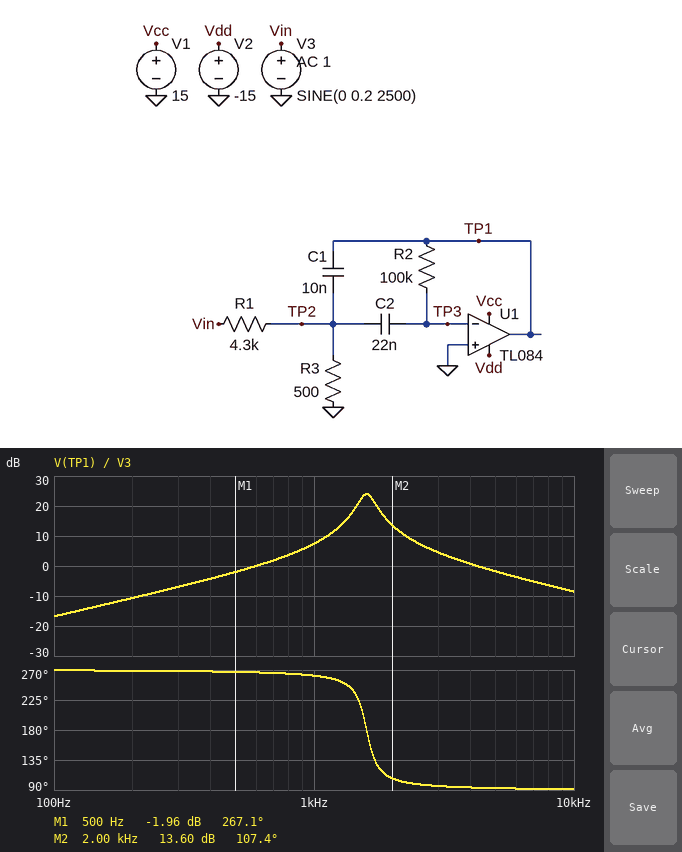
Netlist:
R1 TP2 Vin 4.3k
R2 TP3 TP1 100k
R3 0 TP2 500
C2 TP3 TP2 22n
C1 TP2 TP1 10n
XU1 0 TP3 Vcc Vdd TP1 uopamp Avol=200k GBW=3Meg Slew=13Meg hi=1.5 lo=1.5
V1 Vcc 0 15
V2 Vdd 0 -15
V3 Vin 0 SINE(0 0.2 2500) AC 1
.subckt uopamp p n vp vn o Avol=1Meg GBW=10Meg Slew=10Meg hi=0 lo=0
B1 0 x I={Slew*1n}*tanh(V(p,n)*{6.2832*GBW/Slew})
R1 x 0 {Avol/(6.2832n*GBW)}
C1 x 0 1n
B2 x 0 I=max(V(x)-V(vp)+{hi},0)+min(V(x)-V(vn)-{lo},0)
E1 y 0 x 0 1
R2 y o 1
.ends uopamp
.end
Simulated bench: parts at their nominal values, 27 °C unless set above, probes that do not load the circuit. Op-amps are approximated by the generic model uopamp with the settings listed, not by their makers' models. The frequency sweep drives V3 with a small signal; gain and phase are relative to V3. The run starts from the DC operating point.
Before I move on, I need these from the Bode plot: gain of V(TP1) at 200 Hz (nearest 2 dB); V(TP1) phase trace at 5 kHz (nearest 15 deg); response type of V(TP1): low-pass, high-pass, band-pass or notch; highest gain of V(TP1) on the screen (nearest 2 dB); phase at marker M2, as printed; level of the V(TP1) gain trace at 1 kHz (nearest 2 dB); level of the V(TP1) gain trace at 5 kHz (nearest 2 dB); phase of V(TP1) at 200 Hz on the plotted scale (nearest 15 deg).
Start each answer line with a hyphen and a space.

- -10 dB
- 90 deg
- band-pass
- 24 dB
- 107.4 deg
- 8 dB
- -2 dB
- 270 deg
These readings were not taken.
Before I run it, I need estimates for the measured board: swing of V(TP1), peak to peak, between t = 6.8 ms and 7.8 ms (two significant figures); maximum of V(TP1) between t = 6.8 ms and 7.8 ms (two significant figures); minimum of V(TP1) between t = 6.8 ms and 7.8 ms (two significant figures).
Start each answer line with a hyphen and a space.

- 980 mV
- 490 mV
- -490 mV
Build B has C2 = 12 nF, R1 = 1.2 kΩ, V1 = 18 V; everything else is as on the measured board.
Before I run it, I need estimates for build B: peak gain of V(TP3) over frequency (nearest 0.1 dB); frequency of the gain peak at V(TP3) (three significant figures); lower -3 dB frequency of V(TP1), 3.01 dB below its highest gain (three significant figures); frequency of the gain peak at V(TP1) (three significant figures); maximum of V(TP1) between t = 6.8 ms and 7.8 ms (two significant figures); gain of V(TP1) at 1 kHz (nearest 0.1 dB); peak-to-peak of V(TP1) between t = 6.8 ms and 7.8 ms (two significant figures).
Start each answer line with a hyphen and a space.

- -28.7 dB
- 2.44 kHz
- 2.29 kHz
- 2.43 kHz
- 8.1 V
- 8.5 dB
- 16 V
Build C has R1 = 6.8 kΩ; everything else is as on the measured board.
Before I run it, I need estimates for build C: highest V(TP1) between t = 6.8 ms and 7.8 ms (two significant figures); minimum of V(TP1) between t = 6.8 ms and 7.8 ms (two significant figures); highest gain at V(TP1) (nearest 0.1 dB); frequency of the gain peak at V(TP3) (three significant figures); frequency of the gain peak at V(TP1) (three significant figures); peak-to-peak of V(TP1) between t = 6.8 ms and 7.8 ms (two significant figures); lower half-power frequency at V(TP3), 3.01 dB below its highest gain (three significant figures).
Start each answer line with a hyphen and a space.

- 300 mV
- -300 mV
- 20.1 dB
- 1.57 kHz
- 1.56 kHz
- 600 mV
- 1.47 kHz
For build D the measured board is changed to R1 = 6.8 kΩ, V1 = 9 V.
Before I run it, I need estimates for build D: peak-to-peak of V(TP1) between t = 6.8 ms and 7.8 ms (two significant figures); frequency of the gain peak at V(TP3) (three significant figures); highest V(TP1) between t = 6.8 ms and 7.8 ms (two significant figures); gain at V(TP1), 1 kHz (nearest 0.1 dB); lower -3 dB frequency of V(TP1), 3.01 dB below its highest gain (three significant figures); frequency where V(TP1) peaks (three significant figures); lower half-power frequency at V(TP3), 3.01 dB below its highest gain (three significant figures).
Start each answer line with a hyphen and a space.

- 600 mV
- 1.57 kHz
- 300 mV
- 4.0 dB
- 1.45 kHz
- 1.56 kHz
- 1.47 kHz
